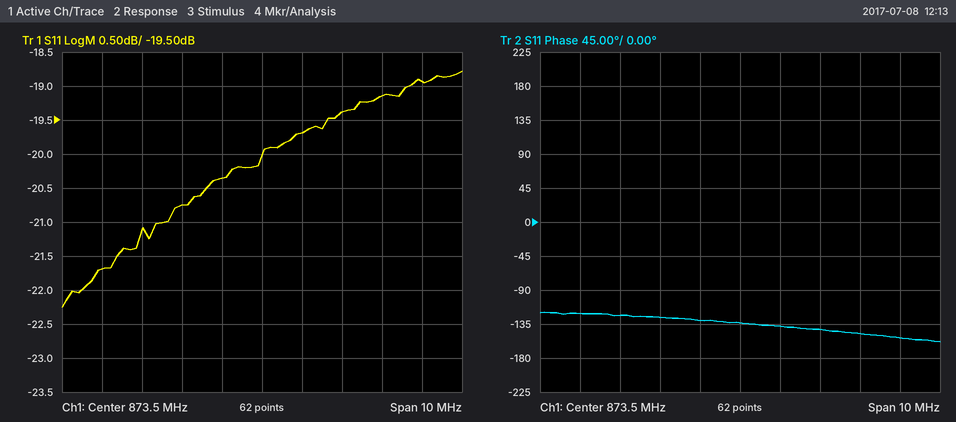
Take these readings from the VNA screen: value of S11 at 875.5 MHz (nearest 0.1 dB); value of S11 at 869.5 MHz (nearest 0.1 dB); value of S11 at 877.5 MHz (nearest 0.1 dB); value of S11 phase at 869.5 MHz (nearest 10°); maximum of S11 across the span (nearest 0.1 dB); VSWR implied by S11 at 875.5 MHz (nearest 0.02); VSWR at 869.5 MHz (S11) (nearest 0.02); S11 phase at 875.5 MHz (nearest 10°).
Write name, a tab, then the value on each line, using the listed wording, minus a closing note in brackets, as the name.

value of S11 at 875.5 MHz	-19.4 dB
value of S11 at 869.5 MHz	-21.7 dB
value of S11 at 877.5 MHz	-18.9 dB
value of S11 phase at 869.5 MHz	-120°
maximum of S11 across the span	-18.8 dB
VSWR implied by S11 at 875.5 MHz	1.24
VSWR at 869.5 MHz (S11)	1.18
S11 phase at 875.5 MHz	-140°
